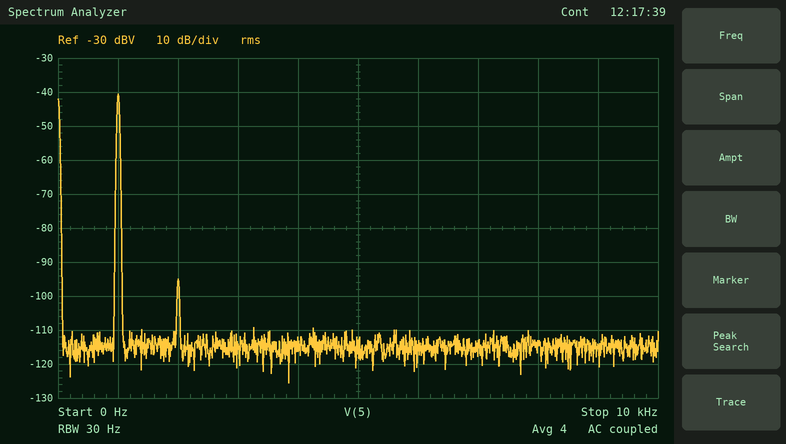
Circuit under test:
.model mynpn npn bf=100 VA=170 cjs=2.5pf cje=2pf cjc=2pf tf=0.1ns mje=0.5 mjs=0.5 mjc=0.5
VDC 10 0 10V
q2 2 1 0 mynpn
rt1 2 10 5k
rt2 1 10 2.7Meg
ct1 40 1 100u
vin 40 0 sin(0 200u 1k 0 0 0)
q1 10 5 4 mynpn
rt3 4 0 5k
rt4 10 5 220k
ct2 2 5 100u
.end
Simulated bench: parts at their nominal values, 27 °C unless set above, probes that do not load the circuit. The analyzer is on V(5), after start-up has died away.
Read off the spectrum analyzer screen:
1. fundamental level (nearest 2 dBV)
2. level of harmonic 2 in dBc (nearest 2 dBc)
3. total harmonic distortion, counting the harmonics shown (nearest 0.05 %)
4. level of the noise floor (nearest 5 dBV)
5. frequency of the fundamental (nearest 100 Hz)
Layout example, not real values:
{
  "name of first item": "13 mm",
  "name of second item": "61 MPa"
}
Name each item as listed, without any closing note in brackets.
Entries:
{
  "fundamental level": "-40 dBV",
  "level of harmonic 2 in dBc": "-54 dBc",
  "total harmonic distortion, counting the harmonics shown": "0.20 %",
  "level of the noise floor": "-115 dBV",
  "frequency of the fundamental": "1.0 kHz"
}
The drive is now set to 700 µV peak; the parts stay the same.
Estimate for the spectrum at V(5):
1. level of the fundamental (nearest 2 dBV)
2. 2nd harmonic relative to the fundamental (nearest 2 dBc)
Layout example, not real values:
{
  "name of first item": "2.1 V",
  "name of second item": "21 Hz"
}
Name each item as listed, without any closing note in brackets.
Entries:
{
  "level of the fundamental": "-30 dBV",
  "2nd harmonic relative to the fundamental": "-44 dBc"
}
